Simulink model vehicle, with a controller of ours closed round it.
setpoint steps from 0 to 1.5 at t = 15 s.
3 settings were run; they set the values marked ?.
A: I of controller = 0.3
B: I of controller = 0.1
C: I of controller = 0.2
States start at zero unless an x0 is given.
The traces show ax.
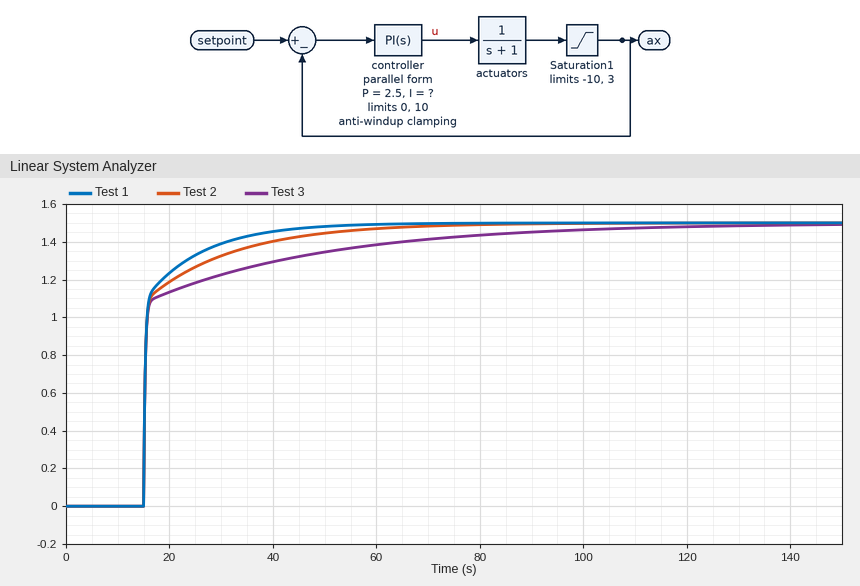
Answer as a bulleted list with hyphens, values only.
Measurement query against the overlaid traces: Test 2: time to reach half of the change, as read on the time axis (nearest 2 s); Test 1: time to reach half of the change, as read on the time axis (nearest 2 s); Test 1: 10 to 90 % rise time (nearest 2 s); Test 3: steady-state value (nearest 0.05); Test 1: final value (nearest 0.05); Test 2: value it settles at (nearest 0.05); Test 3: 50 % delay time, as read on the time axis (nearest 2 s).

- 16 s
- 16 s
- 12 s
- 1.50
- 1.50
- 1.50
- 16 s
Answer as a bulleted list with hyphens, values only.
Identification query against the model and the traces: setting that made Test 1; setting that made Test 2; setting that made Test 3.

- A
- C
- B
